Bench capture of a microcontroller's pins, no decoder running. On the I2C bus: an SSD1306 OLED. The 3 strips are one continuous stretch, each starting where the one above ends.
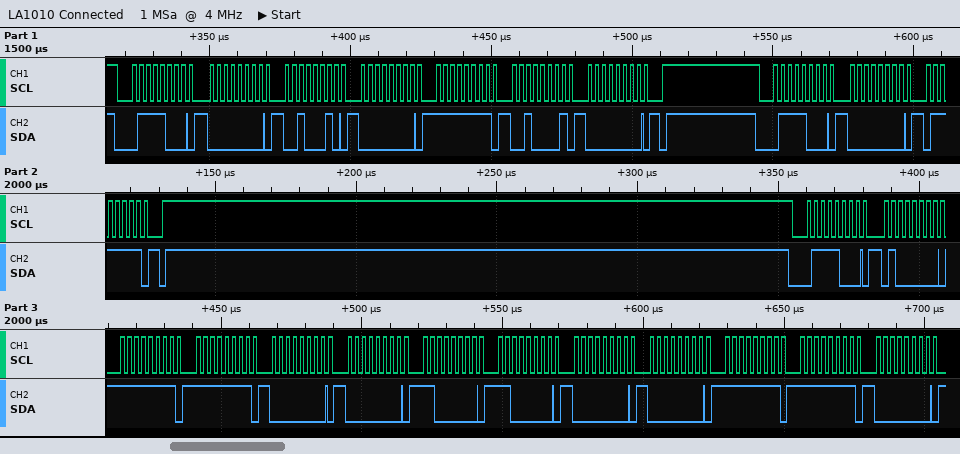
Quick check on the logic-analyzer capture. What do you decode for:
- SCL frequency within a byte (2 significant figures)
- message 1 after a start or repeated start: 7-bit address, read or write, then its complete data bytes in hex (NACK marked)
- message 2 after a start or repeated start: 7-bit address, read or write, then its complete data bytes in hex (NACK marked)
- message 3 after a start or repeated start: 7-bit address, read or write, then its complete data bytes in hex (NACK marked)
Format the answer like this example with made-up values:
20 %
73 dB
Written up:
400 kHz
0x3C write: 00 22 00 FF 21 00
0x3C write: 00 7F
0x3C write: 40 FF FF 00 00 C0 C0 00 00 FF FF 00
